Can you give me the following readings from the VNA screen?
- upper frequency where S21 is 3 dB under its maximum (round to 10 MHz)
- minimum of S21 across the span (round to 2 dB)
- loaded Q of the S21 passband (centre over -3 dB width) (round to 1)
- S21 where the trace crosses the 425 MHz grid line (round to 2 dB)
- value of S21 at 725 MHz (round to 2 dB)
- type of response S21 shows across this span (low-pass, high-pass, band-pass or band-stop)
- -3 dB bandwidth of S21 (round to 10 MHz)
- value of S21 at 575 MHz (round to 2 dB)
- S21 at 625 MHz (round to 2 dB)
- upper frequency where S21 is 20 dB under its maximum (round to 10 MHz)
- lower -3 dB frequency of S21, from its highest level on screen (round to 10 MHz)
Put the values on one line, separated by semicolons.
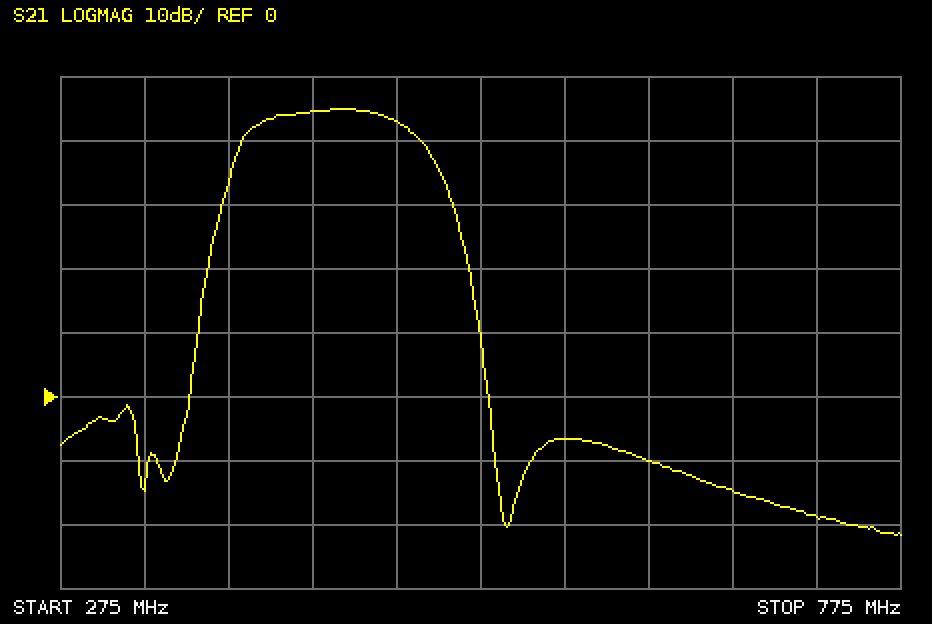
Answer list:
480 MHz; -22 dB; 5; 44 dB; -18 dB; band-pass; 90 MHz; -6 dB; -10 dB; 510 MHz; 390 MHz
